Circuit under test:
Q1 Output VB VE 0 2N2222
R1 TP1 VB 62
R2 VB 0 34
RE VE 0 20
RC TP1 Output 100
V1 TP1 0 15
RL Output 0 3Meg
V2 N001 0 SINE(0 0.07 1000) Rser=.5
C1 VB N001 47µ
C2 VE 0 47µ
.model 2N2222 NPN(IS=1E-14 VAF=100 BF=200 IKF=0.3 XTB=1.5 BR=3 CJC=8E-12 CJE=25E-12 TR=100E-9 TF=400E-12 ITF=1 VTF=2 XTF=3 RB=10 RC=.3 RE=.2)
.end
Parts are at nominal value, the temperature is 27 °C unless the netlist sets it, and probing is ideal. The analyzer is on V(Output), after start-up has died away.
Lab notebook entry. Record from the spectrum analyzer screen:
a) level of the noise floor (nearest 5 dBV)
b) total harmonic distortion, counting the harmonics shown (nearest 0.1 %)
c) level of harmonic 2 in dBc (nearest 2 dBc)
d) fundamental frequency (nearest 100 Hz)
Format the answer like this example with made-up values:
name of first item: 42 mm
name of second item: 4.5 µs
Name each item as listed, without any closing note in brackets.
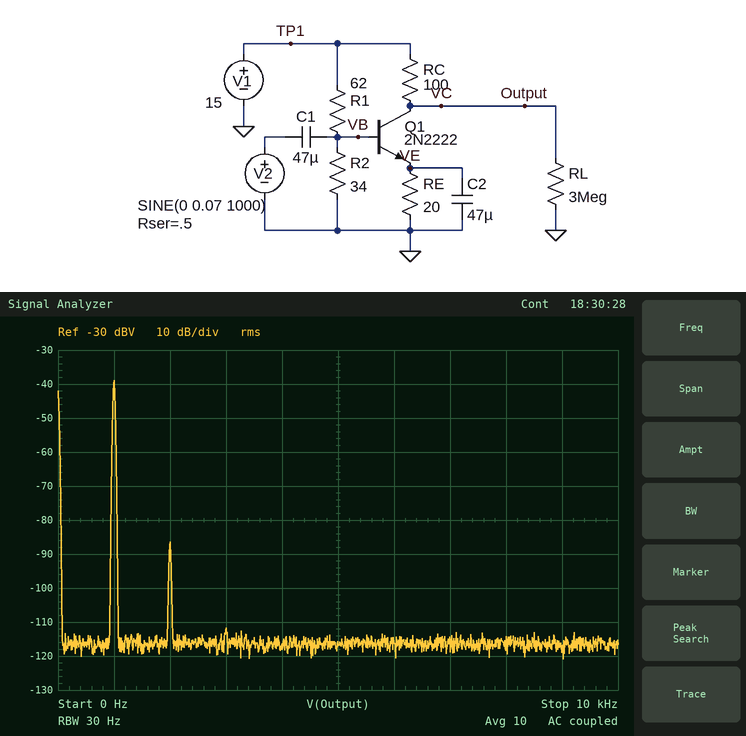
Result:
level of the noise floor: -115 dBV
total harmonic distortion, counting the harmonics shown: 0.4 %
level of harmonic 2 in dBc: -48 dBc
fundamental frequency: 1.0 kHz
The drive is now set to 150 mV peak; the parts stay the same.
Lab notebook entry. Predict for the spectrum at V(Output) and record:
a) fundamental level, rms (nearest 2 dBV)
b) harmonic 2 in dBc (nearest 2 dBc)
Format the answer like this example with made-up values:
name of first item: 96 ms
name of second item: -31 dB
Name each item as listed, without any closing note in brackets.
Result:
fundamental level, rms: -32 dBV
harmonic 2 in dBc: -40 dBc
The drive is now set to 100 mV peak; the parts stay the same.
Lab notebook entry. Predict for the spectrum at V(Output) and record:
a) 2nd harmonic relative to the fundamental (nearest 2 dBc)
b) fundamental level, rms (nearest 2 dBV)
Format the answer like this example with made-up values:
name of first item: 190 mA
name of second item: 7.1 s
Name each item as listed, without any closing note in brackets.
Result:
2nd harmonic relative to the fundamental: -44 dBc
fundamental level, rms: -36 dBV
